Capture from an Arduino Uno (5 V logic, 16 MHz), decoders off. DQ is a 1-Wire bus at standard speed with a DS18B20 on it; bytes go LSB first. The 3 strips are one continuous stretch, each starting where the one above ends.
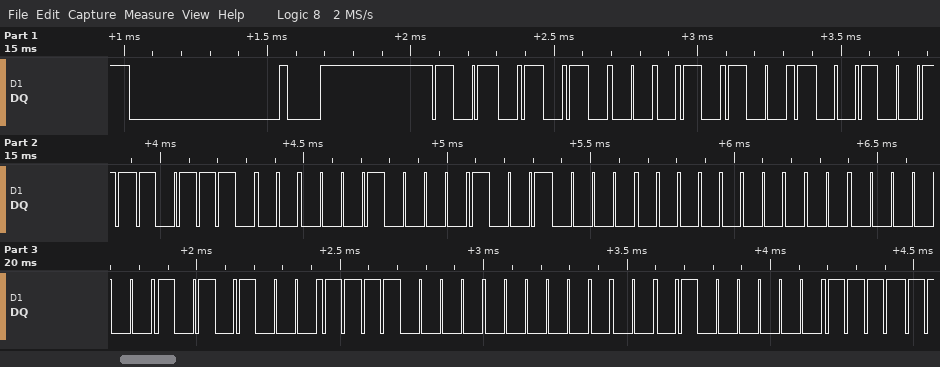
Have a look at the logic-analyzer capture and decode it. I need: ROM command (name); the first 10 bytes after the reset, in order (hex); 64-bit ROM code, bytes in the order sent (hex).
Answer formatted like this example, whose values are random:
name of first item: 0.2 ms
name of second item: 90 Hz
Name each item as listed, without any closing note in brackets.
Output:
ROM command: Match ROM
the first 10 bytes after the reset, in order: 55 28 C9 1D 08 09 00 00 15 0F
64-bit ROM code, bytes in the order sent: 28 C9 1D 08 09 00 00 15
